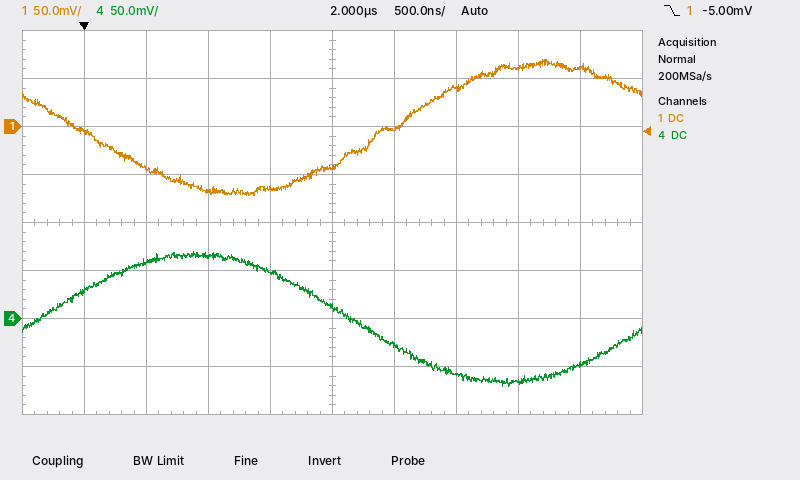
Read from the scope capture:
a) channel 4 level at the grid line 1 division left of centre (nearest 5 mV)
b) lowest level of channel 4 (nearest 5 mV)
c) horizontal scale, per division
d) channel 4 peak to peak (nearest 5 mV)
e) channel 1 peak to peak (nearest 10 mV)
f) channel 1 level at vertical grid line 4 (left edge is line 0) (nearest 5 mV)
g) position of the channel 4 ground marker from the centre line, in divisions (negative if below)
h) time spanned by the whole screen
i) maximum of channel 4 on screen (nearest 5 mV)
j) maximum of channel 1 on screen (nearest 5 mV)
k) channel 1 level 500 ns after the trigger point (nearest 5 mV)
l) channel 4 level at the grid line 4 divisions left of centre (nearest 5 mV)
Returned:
50 mV
-70 mV
500 ns
140 mV
140 mV
-65 mV
-2.0 div
5 µs
70 mV
70 mV
-45 mV
30 mV
